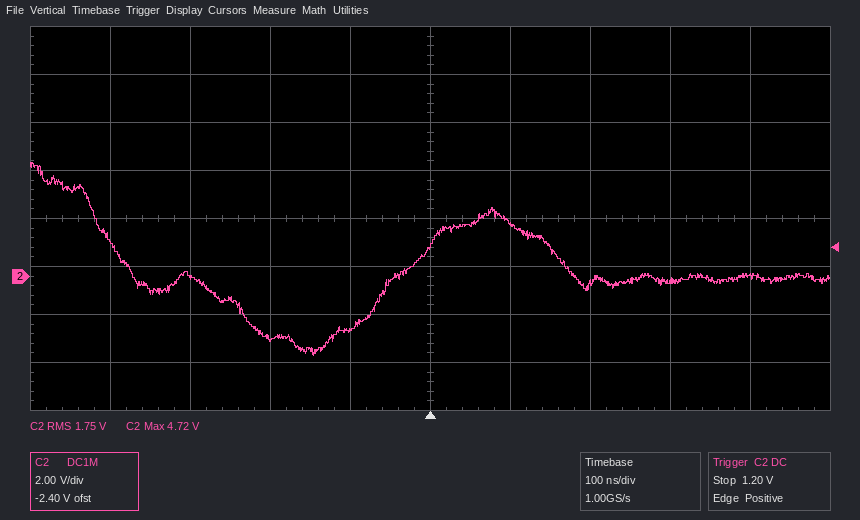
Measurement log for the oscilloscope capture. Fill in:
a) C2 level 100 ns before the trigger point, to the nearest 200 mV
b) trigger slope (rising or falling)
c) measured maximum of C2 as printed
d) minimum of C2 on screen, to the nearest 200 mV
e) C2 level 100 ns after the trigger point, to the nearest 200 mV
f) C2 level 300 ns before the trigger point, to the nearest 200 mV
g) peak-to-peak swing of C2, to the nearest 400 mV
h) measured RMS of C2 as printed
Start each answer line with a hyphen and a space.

- -2.2 V
- rising
- 4.72 V
- -3.4 V
- 2.2 V
- 0.0 V
- 8.0 V
- 1.75 V
